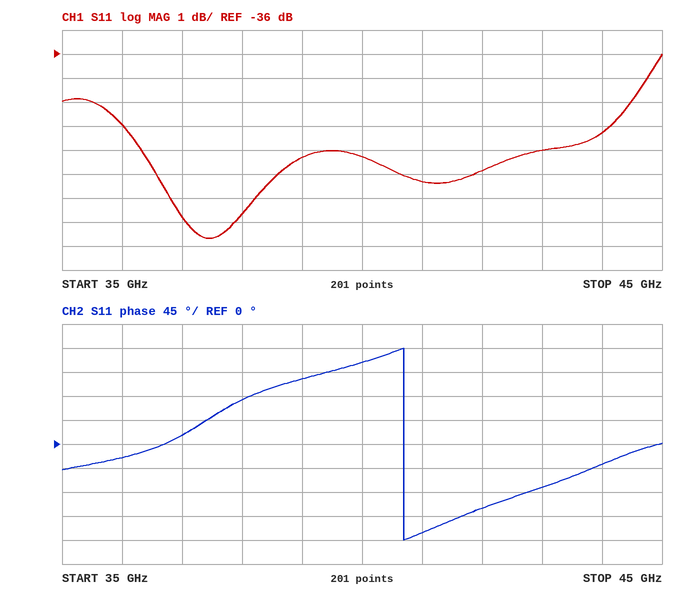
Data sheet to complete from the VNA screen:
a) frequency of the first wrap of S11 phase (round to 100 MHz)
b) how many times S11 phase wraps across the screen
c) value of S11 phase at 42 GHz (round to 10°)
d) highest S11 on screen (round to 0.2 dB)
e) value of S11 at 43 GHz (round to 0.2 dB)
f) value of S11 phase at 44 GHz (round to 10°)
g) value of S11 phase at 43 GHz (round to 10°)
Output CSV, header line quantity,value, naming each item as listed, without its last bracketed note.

quantity,value
frequency of the first wrap of S11 phase,40.7 GHz
how many times S11 phase wraps across the screen,1
value of S11 phase at 42 GHz,-120°
highest S11 on screen,-36.0 dB
value of S11 at 43 GHz,-40.0 dB
value of S11 phase at 44 GHz,-40°
value of S11 phase at 43 GHz,-80°
